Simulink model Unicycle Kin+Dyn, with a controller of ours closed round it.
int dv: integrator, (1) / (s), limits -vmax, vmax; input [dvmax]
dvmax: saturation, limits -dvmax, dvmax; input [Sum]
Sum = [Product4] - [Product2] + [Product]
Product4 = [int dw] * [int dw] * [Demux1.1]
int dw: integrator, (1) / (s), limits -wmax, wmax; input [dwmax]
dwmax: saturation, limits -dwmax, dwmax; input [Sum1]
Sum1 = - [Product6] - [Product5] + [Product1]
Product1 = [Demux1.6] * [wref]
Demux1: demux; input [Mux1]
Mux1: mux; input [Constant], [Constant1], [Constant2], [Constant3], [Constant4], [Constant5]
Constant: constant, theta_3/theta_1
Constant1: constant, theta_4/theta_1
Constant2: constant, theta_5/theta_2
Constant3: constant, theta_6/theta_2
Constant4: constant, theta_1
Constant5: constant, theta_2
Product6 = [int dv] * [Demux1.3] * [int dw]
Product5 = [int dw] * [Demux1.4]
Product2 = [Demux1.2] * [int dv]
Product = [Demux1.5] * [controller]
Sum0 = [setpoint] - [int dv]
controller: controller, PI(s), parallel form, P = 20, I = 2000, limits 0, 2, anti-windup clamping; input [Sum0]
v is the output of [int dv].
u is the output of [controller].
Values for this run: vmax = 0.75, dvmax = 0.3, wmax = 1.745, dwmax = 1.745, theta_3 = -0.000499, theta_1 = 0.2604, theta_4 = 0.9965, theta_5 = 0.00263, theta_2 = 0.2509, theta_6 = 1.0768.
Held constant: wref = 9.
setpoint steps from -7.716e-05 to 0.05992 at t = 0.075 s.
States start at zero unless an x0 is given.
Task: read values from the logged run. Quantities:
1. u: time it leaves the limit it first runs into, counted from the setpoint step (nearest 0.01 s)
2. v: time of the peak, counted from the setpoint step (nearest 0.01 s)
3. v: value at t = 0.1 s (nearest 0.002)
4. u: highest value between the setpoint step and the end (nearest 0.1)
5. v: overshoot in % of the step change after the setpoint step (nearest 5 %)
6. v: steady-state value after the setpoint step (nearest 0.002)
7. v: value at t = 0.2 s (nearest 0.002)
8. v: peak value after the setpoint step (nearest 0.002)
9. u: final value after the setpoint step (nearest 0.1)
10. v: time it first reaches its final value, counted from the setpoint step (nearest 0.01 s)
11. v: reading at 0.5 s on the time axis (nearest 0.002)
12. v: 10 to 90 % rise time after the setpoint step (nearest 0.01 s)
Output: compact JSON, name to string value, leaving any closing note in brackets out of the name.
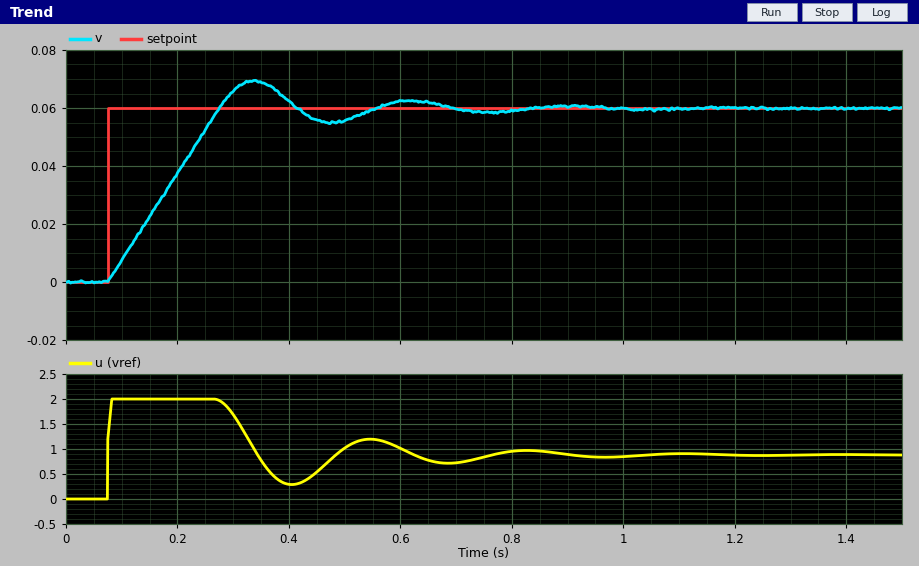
{"u: time it leaves the limit it first runs into, counted from the setpoint step": "0.20 s", "v: time of the peak, counted from the setpoint step": "0.26 s", "v: value at t = 0.1 s": "0.008", "u: highest value between the setpoint step and the end": "2.0", "v: overshoot in % of the step change after the setpoint step": "15 %", "v: steady-state value after the setpoint step": "0.060", "v: value at t = 0.2 s": "0.038", "v: peak value after the setpoint step": "0.070", "u: final value after the setpoint step": "0.9", "v: time it first reaches its final value, counted from the setpoint step": "0.20 s", "v: reading at 0.5 s on the time axis": "0.056", "v: 10 to 90 % rise time after the setpoint step": "0.16 s"}
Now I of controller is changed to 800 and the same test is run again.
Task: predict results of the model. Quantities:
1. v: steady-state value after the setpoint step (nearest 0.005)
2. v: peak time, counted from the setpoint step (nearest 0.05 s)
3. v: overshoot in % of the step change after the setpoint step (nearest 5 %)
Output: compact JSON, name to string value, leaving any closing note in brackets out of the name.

{"v: steady-state value after the setpoint step": "0.060", "v: peak time, counted from the setpoint step": "0.30 s", "v: overshoot in % of the step change after the setpoint step": "20 %"}
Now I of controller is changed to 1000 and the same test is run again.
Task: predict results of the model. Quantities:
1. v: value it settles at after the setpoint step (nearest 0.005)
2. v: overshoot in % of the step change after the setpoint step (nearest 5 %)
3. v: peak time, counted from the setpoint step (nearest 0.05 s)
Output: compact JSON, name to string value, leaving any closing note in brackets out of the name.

{"v: value it settles at after the setpoint step": "0.060", "v: overshoot in % of the step change after the setpoint step": "20 %", "v: peak time, counted from the setpoint step": "0.30 s"}
